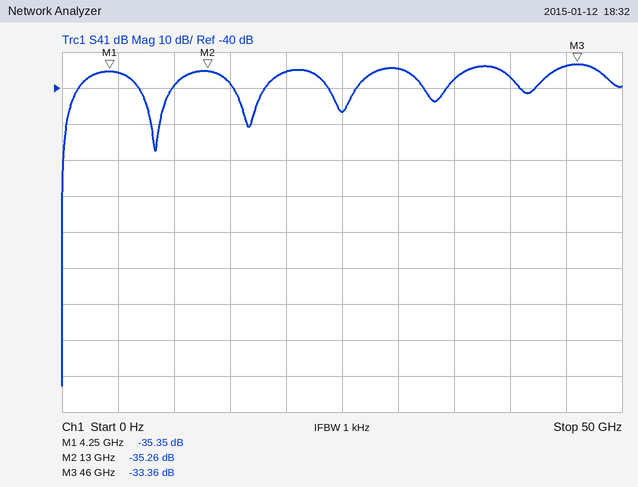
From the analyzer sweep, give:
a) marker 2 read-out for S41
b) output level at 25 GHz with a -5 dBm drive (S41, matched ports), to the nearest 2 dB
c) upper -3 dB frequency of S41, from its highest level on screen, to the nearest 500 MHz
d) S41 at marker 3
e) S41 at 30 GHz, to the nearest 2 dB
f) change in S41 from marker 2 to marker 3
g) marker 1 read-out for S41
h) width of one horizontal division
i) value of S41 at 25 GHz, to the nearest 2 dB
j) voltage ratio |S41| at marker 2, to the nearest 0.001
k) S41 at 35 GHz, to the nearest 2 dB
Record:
-35.26 dB
-52 dBm
48.5 GHz
-33.36 dB
-34 dB
1.90 dB
-35.35 dB
5 GHz
-46 dB
0.017
-38 dB
